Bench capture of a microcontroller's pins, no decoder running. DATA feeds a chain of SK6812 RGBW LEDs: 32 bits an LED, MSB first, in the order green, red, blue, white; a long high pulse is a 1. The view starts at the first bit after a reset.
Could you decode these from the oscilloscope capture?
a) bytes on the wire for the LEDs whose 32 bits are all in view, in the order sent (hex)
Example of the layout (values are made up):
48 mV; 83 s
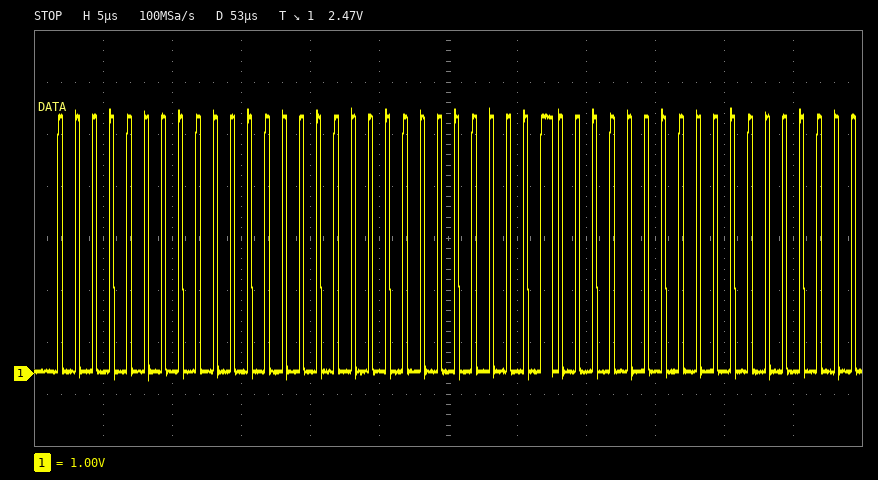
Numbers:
00 00 00 08
